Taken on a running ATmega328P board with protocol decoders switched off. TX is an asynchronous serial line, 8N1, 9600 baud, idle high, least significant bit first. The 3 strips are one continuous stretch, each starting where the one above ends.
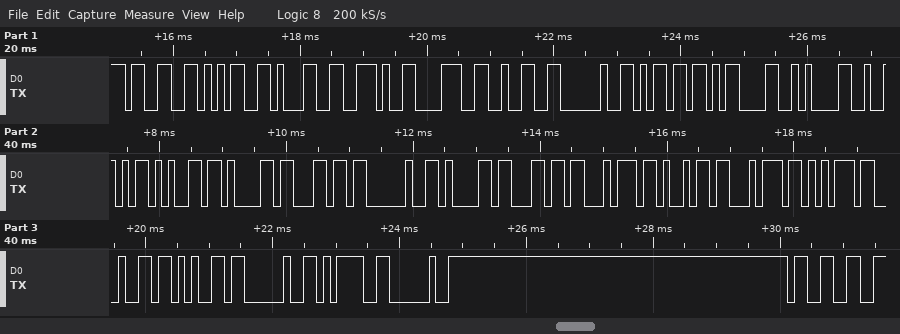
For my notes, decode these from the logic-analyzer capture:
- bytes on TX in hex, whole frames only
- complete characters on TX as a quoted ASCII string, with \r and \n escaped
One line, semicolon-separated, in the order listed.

33 35 31 2E 38 32 20 6D 0D 0A 52 65 61 6C 20 61 6C 74 69 74 75 64 65 20 3D 20 33; "351.82 m\r\nReal altitude = 3"
